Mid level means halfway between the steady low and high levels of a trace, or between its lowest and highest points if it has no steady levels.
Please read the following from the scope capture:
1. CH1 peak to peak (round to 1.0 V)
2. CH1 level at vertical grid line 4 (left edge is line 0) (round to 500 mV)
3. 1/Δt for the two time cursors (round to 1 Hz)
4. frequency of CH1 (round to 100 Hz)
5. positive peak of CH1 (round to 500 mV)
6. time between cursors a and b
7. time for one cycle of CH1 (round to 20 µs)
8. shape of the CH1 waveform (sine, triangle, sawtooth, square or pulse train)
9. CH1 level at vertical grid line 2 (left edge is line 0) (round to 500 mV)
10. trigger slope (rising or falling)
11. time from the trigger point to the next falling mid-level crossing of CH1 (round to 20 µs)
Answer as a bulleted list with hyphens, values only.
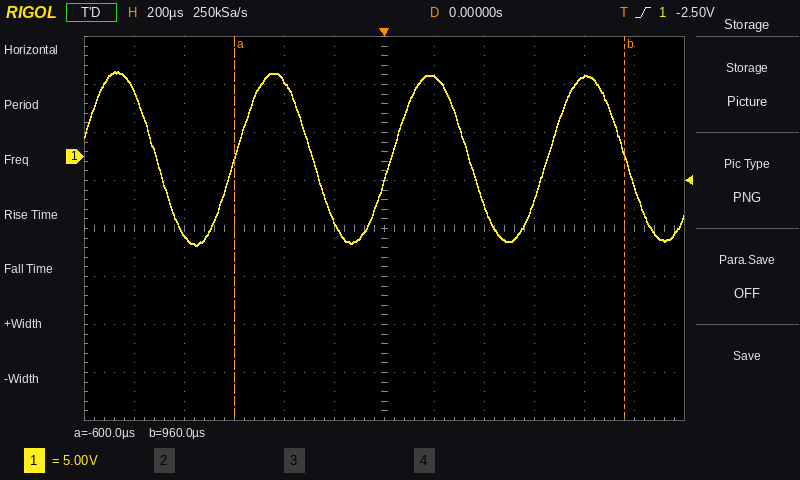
- 18.0 V
- 8.0 V
- 641 Hz
- 1.6 kHz
- 9.0 V
- 1.56 ms
- 620 µs
- sine
- -8.0 V
- rising
- 340 µs
